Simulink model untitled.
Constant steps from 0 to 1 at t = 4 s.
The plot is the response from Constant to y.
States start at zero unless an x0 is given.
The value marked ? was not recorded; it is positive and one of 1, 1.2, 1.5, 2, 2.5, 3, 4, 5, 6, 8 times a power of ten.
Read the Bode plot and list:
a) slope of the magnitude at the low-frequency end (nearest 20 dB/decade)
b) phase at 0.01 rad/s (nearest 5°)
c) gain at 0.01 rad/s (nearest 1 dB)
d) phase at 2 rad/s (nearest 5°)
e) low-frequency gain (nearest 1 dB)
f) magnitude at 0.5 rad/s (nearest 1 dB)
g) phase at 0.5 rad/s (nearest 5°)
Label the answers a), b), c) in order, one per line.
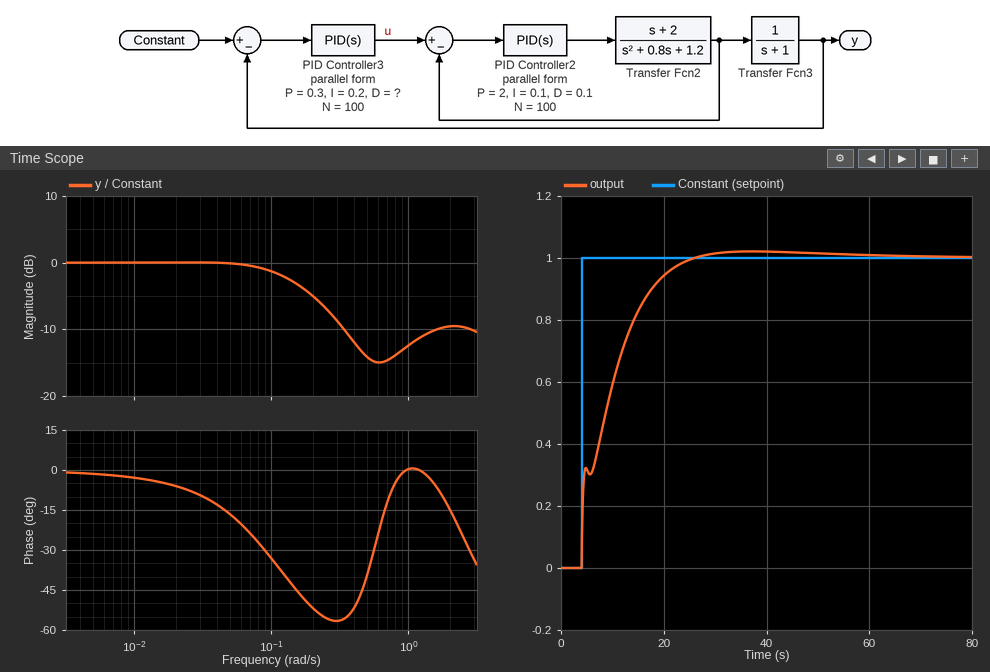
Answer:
a) 0 dB/decade
b) -5°
c) 0 dB
d) -15°
e) 0 dB
f) -14 dB
g) -40°
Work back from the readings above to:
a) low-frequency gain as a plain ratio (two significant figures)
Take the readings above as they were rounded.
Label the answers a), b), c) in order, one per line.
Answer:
a) 1.0
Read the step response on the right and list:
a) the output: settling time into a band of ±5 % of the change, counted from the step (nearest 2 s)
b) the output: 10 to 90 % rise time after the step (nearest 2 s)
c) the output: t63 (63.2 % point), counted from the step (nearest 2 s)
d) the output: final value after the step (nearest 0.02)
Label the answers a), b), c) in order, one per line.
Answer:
a) 16 s
b) 14 s
c) 6 s
d) 1.00
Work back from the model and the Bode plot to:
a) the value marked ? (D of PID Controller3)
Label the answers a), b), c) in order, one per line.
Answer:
a) 0.6
